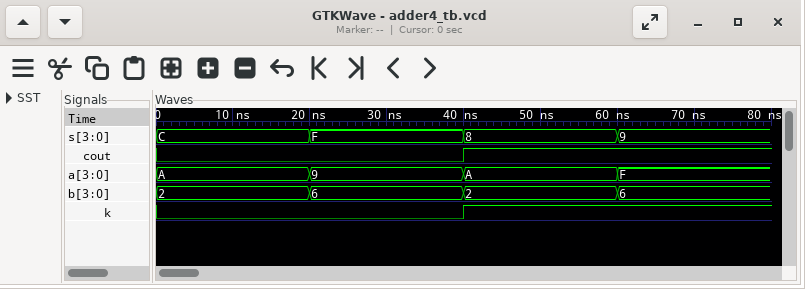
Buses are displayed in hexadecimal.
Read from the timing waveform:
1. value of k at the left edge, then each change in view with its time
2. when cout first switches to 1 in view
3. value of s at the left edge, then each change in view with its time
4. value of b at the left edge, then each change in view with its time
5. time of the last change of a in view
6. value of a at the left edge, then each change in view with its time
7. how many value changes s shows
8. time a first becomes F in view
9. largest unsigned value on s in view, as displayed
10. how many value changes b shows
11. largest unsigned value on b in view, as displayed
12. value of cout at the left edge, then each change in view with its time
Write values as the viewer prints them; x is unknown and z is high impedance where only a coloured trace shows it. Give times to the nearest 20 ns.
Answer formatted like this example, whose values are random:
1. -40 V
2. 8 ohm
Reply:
1. 0, 1 at 40 ns
2. 40 ns
3. C, F at 20 ns, 8 at 40 ns, 9 at 60 ns
4. 2, 6 at 20 ns, 2 at 40 ns, 6 at 60 ns
5. 60 ns
6. A, 9 at 20 ns, A at 40 ns, F at 60 ns
7. 3
8. 60 ns
9. F
10. 3
11. 6
12. 0, 1 at 40 ns
